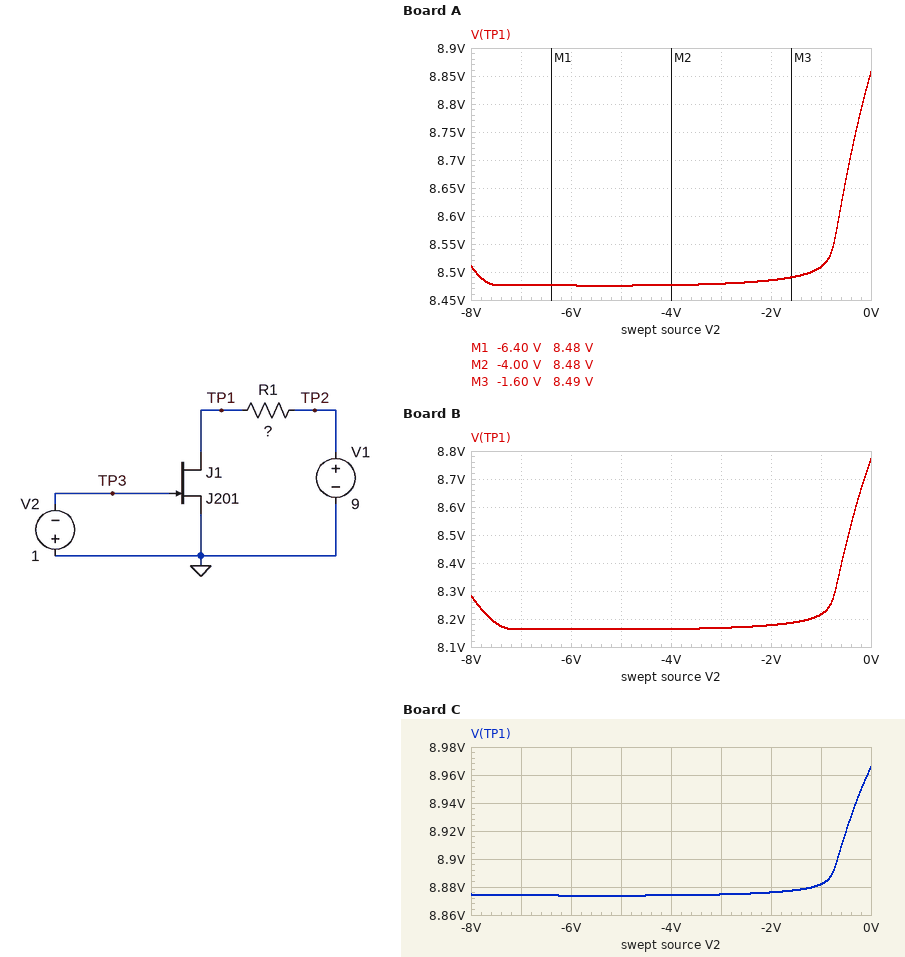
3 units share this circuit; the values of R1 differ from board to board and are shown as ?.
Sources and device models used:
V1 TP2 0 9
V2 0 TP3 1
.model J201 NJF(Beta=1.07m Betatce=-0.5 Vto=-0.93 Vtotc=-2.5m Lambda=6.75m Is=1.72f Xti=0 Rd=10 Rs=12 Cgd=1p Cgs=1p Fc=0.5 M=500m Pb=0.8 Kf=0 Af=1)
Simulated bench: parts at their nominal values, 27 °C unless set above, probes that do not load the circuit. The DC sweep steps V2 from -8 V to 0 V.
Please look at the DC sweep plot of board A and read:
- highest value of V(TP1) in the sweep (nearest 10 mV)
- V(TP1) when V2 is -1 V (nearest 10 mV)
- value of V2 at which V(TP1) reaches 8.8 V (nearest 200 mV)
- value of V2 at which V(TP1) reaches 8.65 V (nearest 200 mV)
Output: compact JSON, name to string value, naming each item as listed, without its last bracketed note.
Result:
{"highest value of V(TP1) in the sweep": "8.86 V", "V(TP1) when V2 is -1 V": "8.51 V", "value of V2 at which V(TP1) reaches 8.8 V": "-200 mV", "value of V2 at which V(TP1) reaches 8.65 V": "-600 mV"}
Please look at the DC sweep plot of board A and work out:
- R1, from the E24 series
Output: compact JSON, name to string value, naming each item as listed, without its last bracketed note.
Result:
{"R1, from the E24 series": "150 Ω"}
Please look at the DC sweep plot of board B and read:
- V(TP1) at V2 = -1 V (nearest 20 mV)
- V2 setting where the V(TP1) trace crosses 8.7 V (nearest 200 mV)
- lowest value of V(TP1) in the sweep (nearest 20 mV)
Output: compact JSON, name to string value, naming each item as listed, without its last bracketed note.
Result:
{"V(TP1) at V2 = -1 V": "8.22 V", "V2 setting where the V(TP1) trace crosses 8.7 V": "-200 mV", "lowest value of V(TP1) in the sweep": "8.16 V"}
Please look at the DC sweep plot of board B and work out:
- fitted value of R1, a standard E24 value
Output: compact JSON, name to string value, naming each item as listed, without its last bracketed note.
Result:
{"fitted value of R1, a standard E24 value": "240 Ω"}
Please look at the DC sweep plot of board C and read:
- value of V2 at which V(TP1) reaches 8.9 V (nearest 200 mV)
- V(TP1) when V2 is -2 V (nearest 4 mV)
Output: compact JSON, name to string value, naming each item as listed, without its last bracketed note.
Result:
{"value of V2 at which V(TP1) reaches 8.9 V": "-600 mV", "V(TP1) when V2 is -2 V": "8.876 V"}
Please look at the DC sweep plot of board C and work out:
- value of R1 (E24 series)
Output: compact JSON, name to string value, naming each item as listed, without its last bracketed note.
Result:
{"value of R1": "36 Ω"}
